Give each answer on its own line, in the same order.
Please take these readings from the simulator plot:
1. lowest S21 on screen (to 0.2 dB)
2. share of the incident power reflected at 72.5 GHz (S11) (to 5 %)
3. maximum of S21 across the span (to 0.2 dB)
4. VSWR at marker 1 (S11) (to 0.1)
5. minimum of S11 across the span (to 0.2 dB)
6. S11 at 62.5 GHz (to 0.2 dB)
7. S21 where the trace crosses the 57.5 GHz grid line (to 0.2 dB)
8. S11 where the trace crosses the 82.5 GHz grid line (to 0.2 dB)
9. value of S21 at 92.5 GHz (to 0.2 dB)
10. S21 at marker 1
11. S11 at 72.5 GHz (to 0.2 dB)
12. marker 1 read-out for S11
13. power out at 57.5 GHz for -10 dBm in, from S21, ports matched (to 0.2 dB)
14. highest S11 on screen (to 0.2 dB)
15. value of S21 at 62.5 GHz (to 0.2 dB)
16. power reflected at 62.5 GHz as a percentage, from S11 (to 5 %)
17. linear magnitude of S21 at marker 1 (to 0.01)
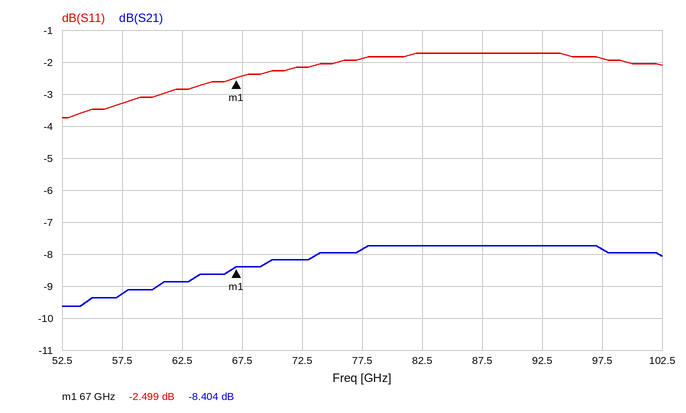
-9.6 dB
60 %
-7.8 dB
7.0
-3.8 dB
-2.8 dB
-9.2 dB
-1.8 dB
-7.8 dB
-8.404 dB
-2.2 dB
-2.499 dB
-19.2 dBm
-1.8 dB
-8.8 dB
50 %
0.38
